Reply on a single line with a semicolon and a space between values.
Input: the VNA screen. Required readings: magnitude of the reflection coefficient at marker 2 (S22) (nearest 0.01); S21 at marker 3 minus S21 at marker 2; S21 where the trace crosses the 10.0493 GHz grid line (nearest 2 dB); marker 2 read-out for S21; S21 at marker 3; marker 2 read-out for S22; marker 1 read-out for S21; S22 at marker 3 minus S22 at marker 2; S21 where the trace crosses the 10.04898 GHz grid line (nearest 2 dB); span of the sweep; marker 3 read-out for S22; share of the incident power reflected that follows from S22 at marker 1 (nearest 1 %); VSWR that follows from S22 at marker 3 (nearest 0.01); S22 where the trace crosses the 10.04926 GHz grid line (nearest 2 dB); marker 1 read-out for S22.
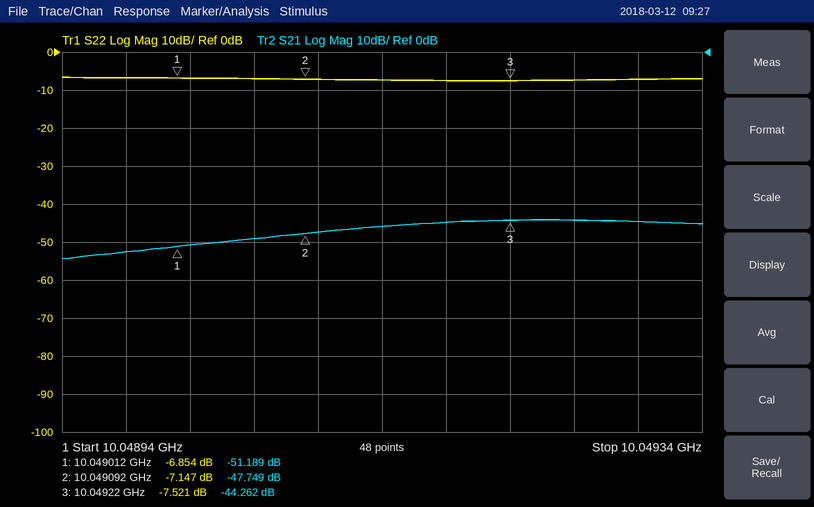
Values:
0.44; 3.487 dB; -44 dB; -47.749 dB; -44.262 dB; -7.147 dB; -51.189 dB; -0.374 dB; -52 dB; 400 kHz; -7.521 dB; 21 %; 2.45; -8 dB; -6.854 dB
